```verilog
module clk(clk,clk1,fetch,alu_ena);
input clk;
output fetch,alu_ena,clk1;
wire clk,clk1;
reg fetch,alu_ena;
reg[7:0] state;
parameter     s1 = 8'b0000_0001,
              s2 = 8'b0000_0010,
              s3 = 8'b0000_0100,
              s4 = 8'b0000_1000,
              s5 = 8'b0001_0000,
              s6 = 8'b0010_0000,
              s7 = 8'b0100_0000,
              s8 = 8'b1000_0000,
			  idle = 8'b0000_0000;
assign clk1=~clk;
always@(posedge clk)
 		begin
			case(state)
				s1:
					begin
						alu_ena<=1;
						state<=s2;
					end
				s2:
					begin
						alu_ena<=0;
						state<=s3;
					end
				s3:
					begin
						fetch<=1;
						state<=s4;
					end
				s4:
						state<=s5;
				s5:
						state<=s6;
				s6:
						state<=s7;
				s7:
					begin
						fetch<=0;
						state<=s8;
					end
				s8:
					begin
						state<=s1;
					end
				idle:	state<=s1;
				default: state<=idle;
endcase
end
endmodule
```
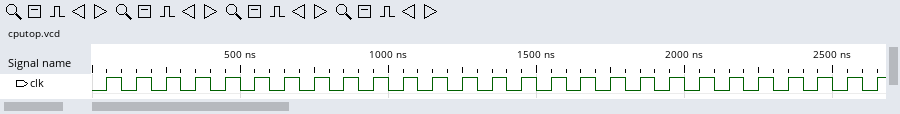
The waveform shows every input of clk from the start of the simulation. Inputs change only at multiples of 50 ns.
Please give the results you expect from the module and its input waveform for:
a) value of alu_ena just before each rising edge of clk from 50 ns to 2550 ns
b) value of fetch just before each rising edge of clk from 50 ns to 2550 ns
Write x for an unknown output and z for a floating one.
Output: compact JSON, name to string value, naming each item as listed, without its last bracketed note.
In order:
{"value of alu_ena just before each rising edge of clk from 50 ns to 2550 ns": "x x x 1 0 0 0 0 0 0 0 1 0 0 0 0 0 0 0 1 0 0 0 0 0 0", "value of fetch just before each rising edge of clk from 50 ns to 2550 ns": "x x x x x 1 1 1 1 0 0 0 0 1 1 1 1 0 0 0 0 1 1 1 1 0"}
